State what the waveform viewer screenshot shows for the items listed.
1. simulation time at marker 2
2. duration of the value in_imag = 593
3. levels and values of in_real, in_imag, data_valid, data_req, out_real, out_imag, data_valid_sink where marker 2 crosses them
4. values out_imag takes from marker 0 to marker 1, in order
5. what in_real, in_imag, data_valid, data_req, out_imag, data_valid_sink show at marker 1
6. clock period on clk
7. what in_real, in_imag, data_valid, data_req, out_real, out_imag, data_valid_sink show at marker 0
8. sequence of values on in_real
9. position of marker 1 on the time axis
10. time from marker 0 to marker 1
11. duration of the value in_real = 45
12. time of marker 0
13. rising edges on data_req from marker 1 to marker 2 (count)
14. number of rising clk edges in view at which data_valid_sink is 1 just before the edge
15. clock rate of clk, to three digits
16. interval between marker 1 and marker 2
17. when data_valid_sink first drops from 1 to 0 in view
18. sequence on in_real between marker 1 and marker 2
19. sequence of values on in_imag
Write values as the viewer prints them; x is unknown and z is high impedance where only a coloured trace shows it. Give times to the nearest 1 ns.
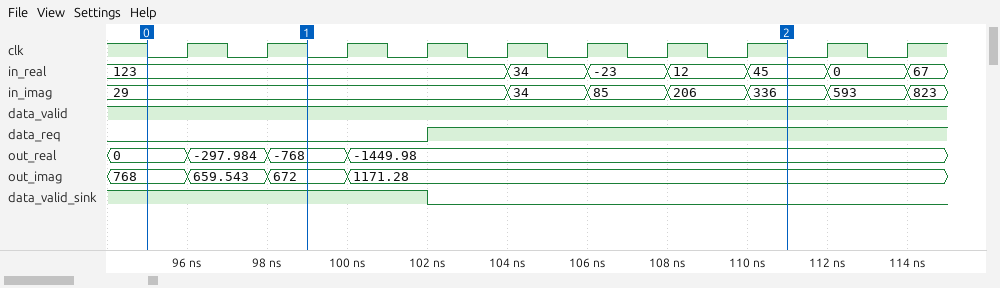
111 ns
2 ns
in_real=45, in_imag=336, data_valid=1, data_req=1, out_real=-1449.98, out_imag=1171.28, data_valid_sink=0
768, 659.543, 672
in_real=123, in_imag=29, data_valid=1, data_req=0, out_imag=672, data_valid_sink=1
2 ns
in_real=123, in_imag=29, data_valid=1, data_req=0, out_real=0, out_imag=768, data_valid_sink=1
123, 34, -23, 12, 45, 0, 67
99 ns
4 ns
2 ns
95 ns
1
4
500 MHz
12 ns
102 ns
123, 34, -23, 12, 45
29, 34, 85, 206, 336, 593, 823
